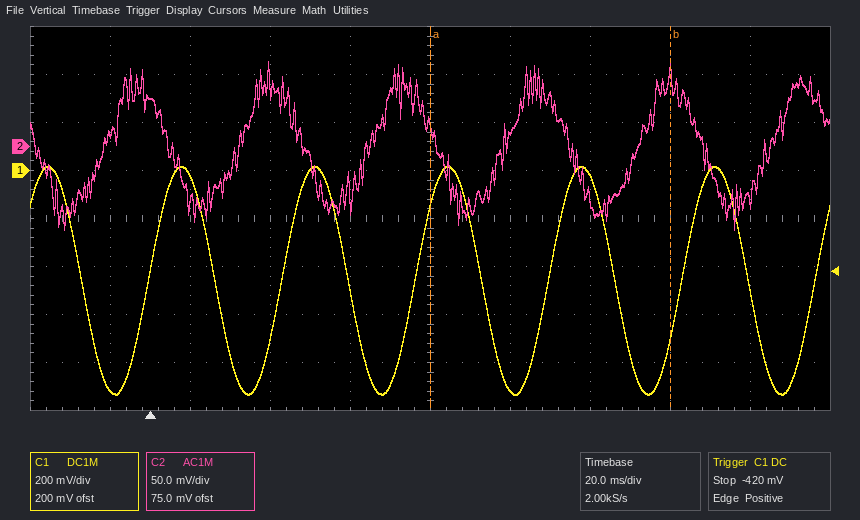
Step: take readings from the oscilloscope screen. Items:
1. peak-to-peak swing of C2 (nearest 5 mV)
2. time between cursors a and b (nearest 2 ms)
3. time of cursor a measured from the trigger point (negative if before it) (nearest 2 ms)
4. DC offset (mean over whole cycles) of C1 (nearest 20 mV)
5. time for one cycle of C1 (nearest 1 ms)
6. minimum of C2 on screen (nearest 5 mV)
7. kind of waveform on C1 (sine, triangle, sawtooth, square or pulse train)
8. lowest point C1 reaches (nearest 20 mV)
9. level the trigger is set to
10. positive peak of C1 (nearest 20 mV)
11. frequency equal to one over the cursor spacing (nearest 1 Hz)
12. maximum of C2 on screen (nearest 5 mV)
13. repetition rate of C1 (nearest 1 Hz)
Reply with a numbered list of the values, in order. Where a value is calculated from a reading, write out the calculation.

1. 90 mV − (-85 mV) = 175 mV
2. 60 ms
3. +70 ms
4. (20 mV + (-940 mV)) / 2 ≈ -460 mV
5. 33 ms
6. -85 mV
7. sine
8. -940 mV
9. -420 mV
10. 20 mV
11. 1 / 60 ms ≈ 17 Hz
12. 90 mV
13. 1 / 33 ms ≈ 30 Hz
